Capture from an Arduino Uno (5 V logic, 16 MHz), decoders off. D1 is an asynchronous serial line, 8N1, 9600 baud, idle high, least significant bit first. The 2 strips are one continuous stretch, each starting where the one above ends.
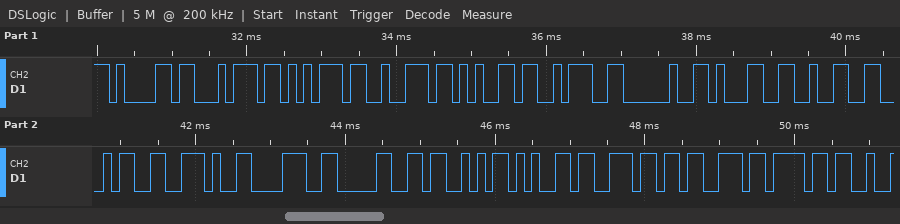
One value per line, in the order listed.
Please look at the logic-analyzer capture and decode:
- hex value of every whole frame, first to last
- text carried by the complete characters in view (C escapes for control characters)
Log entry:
61 74 75 72 65 3A 20 31 32 34 2E 38 30 53 65 6E 73 6F
"ature: 124.80Senso"
